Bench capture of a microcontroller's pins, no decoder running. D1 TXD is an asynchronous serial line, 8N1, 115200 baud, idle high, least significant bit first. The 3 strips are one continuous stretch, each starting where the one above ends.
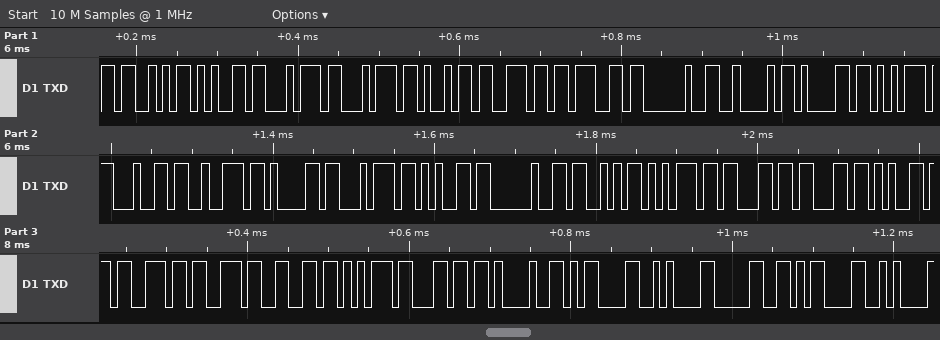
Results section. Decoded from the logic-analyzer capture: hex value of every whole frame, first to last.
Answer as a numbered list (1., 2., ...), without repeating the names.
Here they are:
1. 53 65 74 74 69 6E 67 20 42 61 75 64 72 61 74 65 20 53 75 63 63 65 73 73 66 75 6C 21 0D 0A 30 0D 0A
